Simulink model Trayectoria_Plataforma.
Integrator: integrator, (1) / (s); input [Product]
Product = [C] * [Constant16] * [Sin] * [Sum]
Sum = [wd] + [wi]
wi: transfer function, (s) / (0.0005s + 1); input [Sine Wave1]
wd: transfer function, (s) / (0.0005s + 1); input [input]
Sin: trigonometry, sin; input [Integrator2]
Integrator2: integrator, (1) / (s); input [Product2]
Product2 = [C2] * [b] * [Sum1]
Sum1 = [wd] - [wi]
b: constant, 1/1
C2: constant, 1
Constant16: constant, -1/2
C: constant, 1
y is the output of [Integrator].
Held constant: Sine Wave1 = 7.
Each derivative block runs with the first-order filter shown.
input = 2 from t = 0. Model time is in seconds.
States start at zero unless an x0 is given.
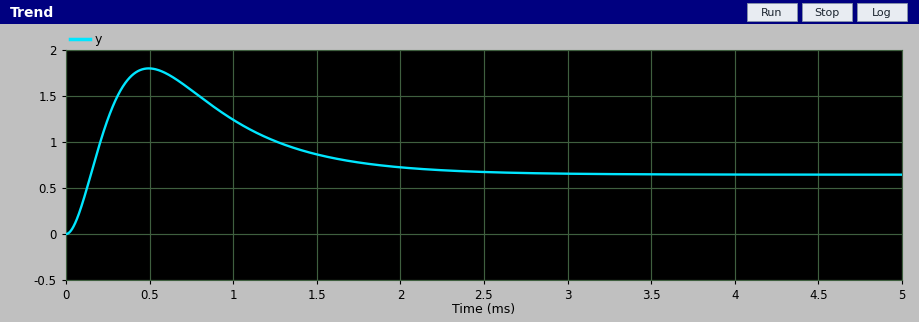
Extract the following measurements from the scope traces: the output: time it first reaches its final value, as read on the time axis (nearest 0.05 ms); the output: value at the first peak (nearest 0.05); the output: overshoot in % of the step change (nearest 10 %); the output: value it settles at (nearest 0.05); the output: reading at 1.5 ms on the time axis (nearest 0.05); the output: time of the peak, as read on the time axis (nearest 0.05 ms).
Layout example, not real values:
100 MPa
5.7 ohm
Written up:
0.15 ms
1.80
180 %
0.65
0.85
0.50 ms
